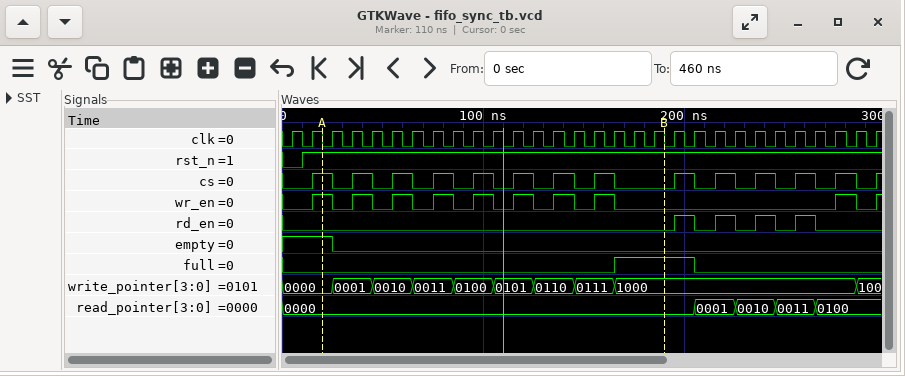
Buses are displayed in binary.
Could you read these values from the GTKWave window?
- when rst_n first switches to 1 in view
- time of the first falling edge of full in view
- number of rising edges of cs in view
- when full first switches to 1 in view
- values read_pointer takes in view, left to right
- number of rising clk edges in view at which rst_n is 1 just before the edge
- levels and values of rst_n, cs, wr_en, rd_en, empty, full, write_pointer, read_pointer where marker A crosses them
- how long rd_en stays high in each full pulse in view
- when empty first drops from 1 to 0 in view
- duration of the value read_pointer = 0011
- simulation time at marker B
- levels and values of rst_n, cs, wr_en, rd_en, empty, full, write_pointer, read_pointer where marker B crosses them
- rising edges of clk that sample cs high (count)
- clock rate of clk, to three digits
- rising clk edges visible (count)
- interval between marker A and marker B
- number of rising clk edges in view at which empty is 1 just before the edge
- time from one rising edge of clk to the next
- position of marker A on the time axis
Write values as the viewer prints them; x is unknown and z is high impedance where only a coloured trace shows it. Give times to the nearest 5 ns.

10 ns
205 ns
14
165 ns
0000, 0001, 0010, 0011, 0100
29
rst_n=1, cs=1, wr_en=1, rd_en=0, empty=1, full=0, write_pointer=0000, read_pointer=0000
10 ns, 10 ns, 10 ns, 10 ns
25 ns
20 ns
190 ns
rst_n=1, cs=0, wr_en=0, rd_en=0, empty=0, full=1, write_pointer=1000, read_pointer=0000
13
100 MHz
30
170 ns
3
10 ns
20 ns
